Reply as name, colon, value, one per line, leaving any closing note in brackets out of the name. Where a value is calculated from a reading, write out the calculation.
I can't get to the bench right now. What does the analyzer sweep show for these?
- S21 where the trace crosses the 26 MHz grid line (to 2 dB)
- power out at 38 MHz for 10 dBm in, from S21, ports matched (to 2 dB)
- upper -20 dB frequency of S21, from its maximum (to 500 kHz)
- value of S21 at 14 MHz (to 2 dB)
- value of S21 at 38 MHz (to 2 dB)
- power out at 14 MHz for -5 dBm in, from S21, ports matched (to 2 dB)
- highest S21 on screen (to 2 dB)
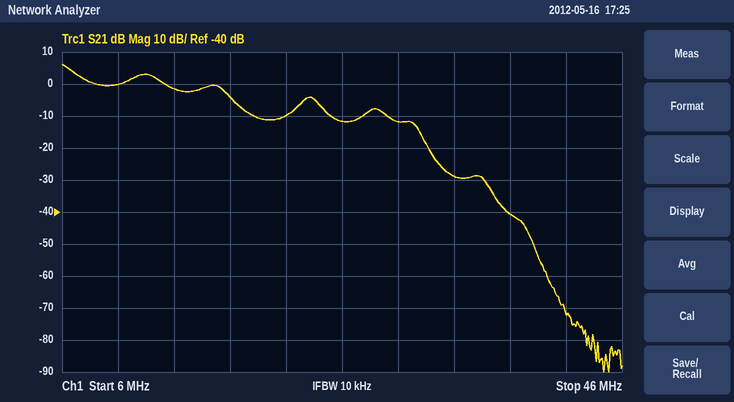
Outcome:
S21 where the trace crosses the 26 MHz grid line: -12 dB
power out at 38 MHz for 10 dBm in, from S21, ports matched: 10 dBm + (-40 dB) = -30 dBm
upper -20 dB frequency of S21, from its maximum: 31.5 MHz
value of S21 at 14 MHz: -2 dB
value of S21 at 38 MHz: -40 dB
power out at 14 MHz for -5 dBm in, from S21, ports matched: -5 dBm + (-2 dB) = -6 dBm
highest S21 on screen: 6 dB
